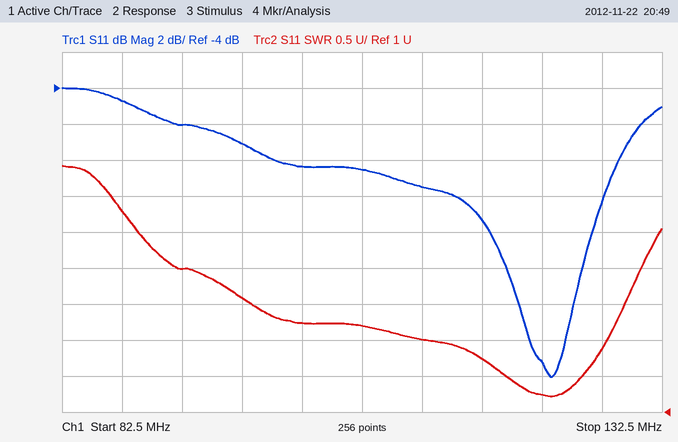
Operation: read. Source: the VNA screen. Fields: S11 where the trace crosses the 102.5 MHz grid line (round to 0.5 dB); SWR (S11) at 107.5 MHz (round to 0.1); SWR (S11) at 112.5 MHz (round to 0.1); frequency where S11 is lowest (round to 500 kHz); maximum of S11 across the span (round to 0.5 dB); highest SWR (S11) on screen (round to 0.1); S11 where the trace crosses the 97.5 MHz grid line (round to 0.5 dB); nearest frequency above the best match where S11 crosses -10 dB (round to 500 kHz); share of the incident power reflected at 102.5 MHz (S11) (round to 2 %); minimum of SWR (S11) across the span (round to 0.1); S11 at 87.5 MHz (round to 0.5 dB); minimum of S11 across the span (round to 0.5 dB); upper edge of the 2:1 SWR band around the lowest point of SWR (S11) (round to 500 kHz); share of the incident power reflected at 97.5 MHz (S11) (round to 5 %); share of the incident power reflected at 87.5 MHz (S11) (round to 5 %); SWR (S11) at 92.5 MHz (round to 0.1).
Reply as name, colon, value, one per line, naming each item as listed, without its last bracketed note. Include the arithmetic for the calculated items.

S11 where the trace crosses the 102.5 MHz grid line: -8.5 dB
SWR (S11) at 107.5 MHz: 2.2
SWR (S11) at 112.5 MHz: 2.0
frequency where S11 is lowest: 123.0 MHz
maximum of S11 across the span: -4.0 dB
highest SWR (S11) on screen: 4.4
S11 where the trace crosses the 97.5 MHz grid line: -7.0 dB
nearest frequency above the best match where S11 crosses -10 dB: 127.5 MHz
share of the incident power reflected at 102.5 MHz (S11): 10^(-8.5/10) ≈ 14 %
minimum of SWR (S11) across the span: 1.2
S11 at 87.5 MHz: -4.5 dB
minimum of S11 across the span: -20.0 dB
upper edge of the 2:1 SWR band around the lowest point of SWR (S11): 128.0 MHz
share of the incident power reflected at 97.5 MHz (S11): 10^(-7/10) ≈ 20 %
share of the incident power reflected at 87.5 MHz (S11): 10^(-4.5/10) ≈ 35 %
SWR (S11) at 92.5 MHz: 3.0
